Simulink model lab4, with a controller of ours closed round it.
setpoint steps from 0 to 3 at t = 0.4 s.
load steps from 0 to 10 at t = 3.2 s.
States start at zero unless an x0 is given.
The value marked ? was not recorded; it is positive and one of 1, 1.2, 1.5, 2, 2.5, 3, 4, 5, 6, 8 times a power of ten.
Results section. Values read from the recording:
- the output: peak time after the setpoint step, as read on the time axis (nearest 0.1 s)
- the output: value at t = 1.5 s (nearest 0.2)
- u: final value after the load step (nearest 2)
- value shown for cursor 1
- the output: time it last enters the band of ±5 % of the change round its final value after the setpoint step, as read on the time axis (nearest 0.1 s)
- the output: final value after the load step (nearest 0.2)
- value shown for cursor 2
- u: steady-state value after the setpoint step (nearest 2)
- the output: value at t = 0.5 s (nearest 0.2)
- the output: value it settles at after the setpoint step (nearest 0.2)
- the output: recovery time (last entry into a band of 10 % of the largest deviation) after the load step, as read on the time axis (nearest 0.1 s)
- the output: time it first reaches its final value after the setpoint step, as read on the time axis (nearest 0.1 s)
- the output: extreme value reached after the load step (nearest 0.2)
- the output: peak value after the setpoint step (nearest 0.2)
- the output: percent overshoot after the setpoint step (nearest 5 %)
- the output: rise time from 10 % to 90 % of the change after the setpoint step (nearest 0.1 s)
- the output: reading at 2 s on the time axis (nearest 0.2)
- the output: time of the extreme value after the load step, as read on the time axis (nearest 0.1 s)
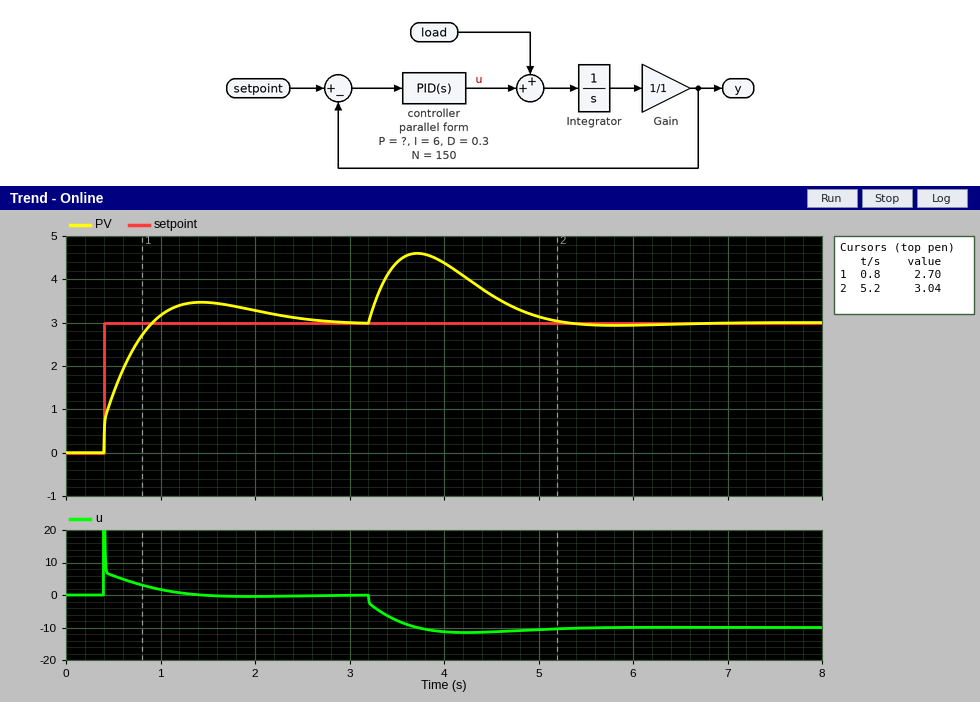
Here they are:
1.4 s
3.4
-10
2.70
2.3 s
3.0
3.04
0
1.4
3.0
5.0 s
0.9 s
4.6
3.4
15 %
0.4 s
3.2
3.7 s
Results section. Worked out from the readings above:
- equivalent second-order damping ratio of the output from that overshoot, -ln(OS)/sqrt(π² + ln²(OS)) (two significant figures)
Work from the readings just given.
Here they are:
0.52
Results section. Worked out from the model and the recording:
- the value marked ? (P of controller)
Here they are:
4
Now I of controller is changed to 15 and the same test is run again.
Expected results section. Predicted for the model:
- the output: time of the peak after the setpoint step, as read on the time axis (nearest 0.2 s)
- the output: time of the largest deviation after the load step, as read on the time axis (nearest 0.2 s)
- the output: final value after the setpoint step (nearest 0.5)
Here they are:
1.2 s
3.6 s
3.0
